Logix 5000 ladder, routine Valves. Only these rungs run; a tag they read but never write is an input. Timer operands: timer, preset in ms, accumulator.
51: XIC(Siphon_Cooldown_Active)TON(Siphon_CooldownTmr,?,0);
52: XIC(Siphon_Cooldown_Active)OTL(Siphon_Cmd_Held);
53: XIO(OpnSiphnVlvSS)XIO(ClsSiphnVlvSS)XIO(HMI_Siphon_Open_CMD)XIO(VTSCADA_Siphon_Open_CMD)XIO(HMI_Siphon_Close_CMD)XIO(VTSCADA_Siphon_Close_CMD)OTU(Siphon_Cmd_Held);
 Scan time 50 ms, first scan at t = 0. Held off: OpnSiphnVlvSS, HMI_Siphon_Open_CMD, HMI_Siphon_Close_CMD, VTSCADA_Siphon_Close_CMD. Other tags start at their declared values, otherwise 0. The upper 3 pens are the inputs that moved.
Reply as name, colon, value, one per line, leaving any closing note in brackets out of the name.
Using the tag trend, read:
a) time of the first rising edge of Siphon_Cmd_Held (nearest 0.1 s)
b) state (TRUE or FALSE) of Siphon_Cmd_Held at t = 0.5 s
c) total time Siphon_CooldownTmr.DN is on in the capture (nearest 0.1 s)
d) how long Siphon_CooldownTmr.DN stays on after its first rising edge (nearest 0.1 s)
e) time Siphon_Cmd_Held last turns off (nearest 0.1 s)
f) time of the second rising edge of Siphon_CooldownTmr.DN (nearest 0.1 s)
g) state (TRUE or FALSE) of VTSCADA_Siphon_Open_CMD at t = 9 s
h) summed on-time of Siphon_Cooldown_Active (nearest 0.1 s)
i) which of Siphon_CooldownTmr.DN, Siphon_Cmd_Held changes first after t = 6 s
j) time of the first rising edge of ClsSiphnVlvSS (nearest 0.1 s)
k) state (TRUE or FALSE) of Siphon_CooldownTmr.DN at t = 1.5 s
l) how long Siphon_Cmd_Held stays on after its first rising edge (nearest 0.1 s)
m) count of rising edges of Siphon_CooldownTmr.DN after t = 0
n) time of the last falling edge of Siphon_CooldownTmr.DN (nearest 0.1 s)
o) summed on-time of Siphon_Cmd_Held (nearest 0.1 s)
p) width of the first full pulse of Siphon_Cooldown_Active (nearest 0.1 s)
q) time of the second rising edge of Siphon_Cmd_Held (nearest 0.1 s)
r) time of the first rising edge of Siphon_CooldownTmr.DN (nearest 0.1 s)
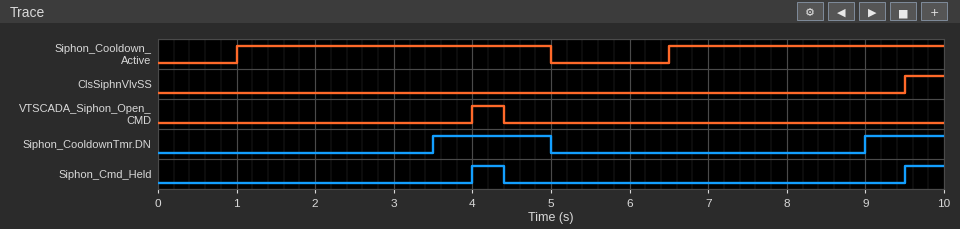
time of the first rising edge of Siphon_Cmd_Held: 4.0 s
state (TRUE or FALSE) of Siphon_Cmd_Held at t = 0.5 s: FALSE
total time Siphon_CooldownTmr.DN is on in the capture: 2.5 s
how long Siphon_CooldownTmr.DN stays on after its first rising edge: 1.5 s
time Siphon_Cmd_Held last turns off: 4.4 s
time of the second rising edge of Siphon_CooldownTmr.DN: 9.0 s
state (TRUE or FALSE) of VTSCADA_Siphon_Open_CMD at t = 9 s: FALSE
summed on-time of Siphon_Cooldown_Active: 7.5 s
which of Siphon_CooldownTmr.DN, Siphon_Cmd_Held changes first after t = 6 s: Siphon_CooldownTmr.DN
time of the first rising edge of ClsSiphnVlvSS: 9.5 s
state (TRUE or FALSE) of Siphon_CooldownTmr.DN at t = 1.5 s: FALSE
how long Siphon_Cmd_Held stays on after its first rising edge: 0.4 s
count of rising edges of Siphon_CooldownTmr.DN after t = 0: 2
time of the last falling edge of Siphon_CooldownTmr.DN: 5.0 s
summed on-time of Siphon_Cmd_Held: 0.9 s
width of the first full pulse of Siphon_Cooldown_Active: 4.0 s
time of the second rising edge of Siphon_Cmd_Held: 9.5 s
time of the first rising edge of Siphon_CooldownTmr.DN: 3.5 s
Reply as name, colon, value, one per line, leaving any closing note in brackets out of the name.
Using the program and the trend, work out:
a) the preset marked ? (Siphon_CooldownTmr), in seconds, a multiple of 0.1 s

the preset marked ? (Siphon_CooldownTmr), in seconds, a multiple of 0.1 s: 2.5 s
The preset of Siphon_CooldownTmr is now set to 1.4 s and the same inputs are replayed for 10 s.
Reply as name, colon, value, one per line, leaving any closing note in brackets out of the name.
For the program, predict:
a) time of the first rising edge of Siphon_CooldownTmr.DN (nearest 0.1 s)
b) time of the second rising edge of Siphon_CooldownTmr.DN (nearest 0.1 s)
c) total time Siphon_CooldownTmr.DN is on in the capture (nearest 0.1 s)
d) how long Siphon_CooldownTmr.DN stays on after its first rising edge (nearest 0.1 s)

time of the first rising edge of Siphon_CooldownTmr.DN: 2.4 s
time of the second rising edge of Siphon_CooldownTmr.DN: 7.9 s
total time Siphon_CooldownTmr.DN is on in the capture: 4.7 s
how long Siphon_CooldownTmr.DN stays on after its first rising edge: 2.6 s
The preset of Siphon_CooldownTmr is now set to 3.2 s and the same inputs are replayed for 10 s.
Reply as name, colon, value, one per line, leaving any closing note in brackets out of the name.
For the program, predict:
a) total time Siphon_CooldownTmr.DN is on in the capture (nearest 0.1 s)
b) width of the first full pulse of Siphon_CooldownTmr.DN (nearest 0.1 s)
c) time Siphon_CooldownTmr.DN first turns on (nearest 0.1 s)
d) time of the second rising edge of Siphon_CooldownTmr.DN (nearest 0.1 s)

total time Siphon_CooldownTmr.DN is on in the capture: 1.1 s
width of the first full pulse of Siphon_CooldownTmr.DN: 0.8 s
time Siphon_CooldownTmr.DN first turns on: 4.2 s
time of the second rising edge of Siphon_CooldownTmr.DN: 9.7 s
